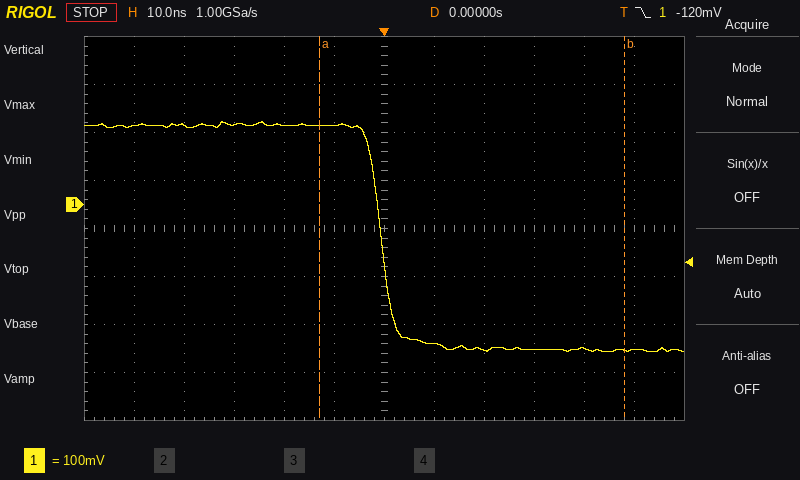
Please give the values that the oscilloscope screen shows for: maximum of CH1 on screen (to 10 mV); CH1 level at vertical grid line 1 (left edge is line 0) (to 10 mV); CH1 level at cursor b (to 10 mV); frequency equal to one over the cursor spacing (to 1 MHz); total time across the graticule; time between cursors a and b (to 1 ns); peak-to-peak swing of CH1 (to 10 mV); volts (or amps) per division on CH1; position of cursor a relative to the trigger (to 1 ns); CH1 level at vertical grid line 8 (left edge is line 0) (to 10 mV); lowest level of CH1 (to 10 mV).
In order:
170 mV
160 mV
-300 mV
16 MHz
120 ns
61 ns
480 mV
100 mV
-13 ns
-300 mV
-310 mV
